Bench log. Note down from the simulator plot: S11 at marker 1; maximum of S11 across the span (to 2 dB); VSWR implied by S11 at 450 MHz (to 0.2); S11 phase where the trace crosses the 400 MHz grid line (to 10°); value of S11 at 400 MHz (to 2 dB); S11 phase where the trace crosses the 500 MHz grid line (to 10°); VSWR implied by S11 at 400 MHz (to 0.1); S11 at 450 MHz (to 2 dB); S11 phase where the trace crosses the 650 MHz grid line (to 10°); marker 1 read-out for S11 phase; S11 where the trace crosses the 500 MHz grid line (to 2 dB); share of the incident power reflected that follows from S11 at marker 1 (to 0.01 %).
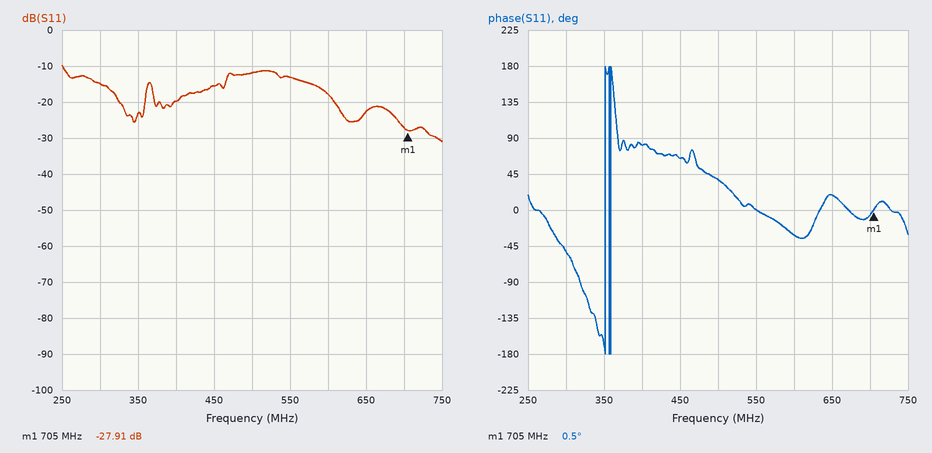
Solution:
-27.91 dB
-10 dB
1.4
80°
-20 dB
40°
1.2
-16 dB
20°
0.5°
-12 dB
0.16 %
